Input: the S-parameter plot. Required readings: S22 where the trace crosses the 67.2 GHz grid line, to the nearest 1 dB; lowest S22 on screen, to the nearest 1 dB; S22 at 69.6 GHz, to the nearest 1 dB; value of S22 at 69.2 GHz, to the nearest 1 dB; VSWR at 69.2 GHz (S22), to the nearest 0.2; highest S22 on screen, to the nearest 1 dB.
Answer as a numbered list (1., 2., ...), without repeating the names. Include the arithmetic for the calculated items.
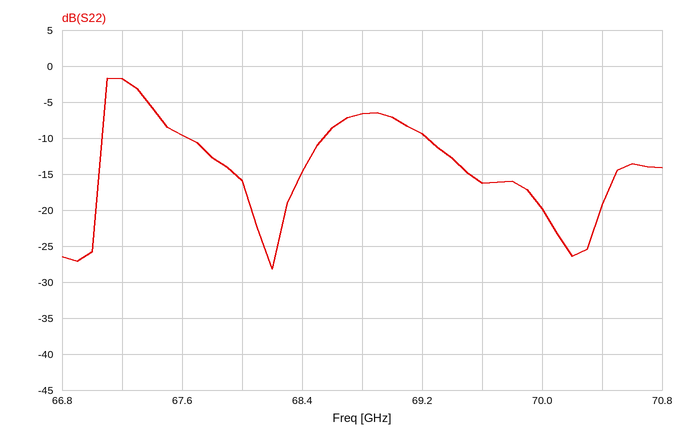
1. -2 dB
2. -28 dB
3. -16 dB
4. -9 dB
5. |Γ| = 10^(-9/20) = 0.3548; VSWR = (1 + 0.3548)/(1 − 0.3548) ≈ 2.10, so 2.0 to the nearest 0.2
6. -2 dB
